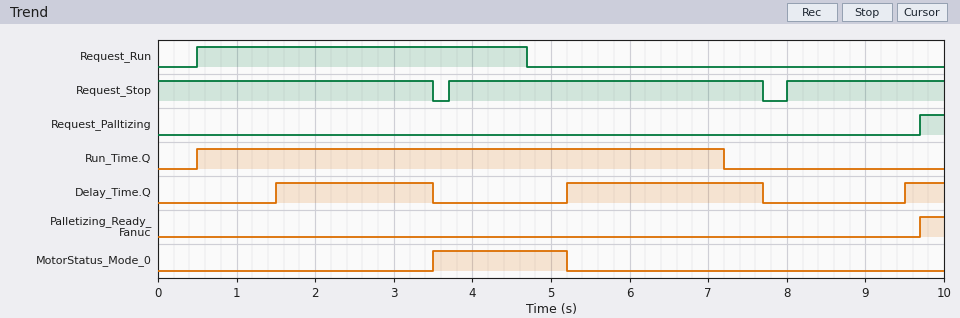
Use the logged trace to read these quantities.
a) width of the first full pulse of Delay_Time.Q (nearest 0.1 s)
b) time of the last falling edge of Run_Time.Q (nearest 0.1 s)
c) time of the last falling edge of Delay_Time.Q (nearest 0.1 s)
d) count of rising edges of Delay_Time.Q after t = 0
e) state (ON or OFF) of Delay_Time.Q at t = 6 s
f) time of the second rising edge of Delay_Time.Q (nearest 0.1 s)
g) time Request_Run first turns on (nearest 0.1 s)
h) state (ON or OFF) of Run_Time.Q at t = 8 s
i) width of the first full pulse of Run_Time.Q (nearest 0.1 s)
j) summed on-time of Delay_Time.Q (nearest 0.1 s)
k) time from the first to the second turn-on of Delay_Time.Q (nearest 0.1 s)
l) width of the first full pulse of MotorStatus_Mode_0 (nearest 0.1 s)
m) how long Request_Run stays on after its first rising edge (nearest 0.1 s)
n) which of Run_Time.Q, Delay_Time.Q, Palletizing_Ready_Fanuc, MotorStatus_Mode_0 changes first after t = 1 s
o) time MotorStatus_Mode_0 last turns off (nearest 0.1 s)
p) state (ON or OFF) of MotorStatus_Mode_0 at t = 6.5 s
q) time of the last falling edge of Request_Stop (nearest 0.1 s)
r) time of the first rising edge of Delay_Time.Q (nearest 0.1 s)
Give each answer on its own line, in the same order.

2.0 s
7.2 s
7.7 s
3
ON
5.2 s
0.5 s
OFF
6.7 s
5.0 s
3.7 s
1.7 s
4.2 s
Delay_Time.Q
5.2 s
OFF
7.7 s
1.5 s
